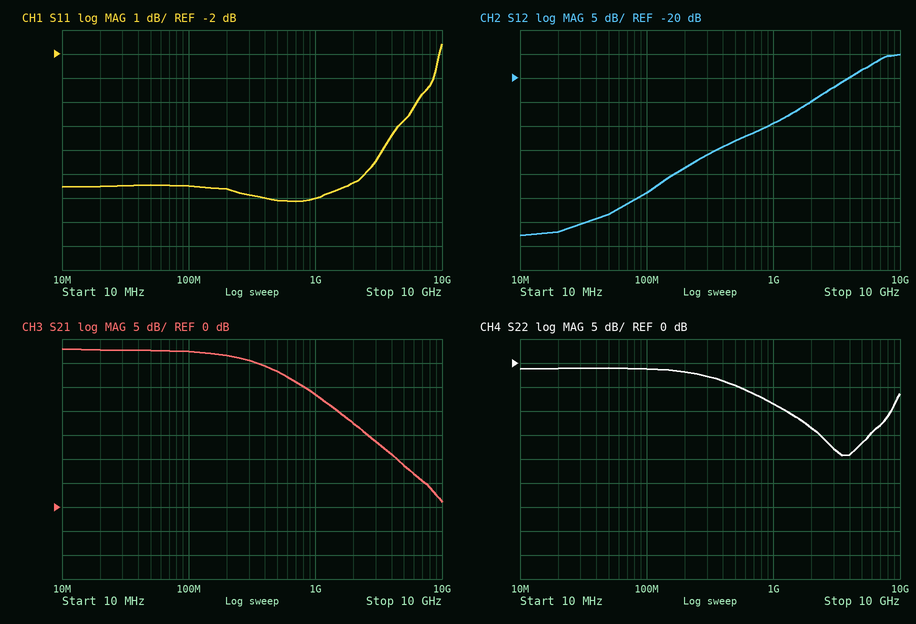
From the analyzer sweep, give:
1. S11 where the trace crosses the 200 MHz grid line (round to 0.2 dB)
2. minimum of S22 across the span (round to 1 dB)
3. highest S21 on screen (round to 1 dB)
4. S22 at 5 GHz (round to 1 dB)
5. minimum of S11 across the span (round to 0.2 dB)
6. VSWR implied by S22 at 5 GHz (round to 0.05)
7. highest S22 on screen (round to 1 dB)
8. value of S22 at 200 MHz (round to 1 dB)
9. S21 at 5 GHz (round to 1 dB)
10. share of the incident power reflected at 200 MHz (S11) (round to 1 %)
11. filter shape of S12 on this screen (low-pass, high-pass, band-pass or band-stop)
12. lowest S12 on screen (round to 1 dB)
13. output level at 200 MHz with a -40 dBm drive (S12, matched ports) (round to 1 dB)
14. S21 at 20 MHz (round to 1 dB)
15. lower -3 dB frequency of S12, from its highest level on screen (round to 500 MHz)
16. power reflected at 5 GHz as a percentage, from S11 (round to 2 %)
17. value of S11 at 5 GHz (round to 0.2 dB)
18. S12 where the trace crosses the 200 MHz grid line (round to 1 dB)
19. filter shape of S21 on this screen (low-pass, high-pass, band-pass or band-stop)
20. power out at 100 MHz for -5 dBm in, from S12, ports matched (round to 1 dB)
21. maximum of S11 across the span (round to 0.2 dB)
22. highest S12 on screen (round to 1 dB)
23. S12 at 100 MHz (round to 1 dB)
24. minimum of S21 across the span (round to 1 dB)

-7.6 dB
-19 dB
33 dB
-17 dB
-8.2 dB
1.35
-1 dB
-2 dB
9 dB
17 %
high-pass
-53 dB
-79 dBm
33 dB
5.0 GHz
34 %
-4.8 dB
-39 dB
low-pass
-49 dBm
-1.6 dB
-15 dB
-44 dB
1 dB
